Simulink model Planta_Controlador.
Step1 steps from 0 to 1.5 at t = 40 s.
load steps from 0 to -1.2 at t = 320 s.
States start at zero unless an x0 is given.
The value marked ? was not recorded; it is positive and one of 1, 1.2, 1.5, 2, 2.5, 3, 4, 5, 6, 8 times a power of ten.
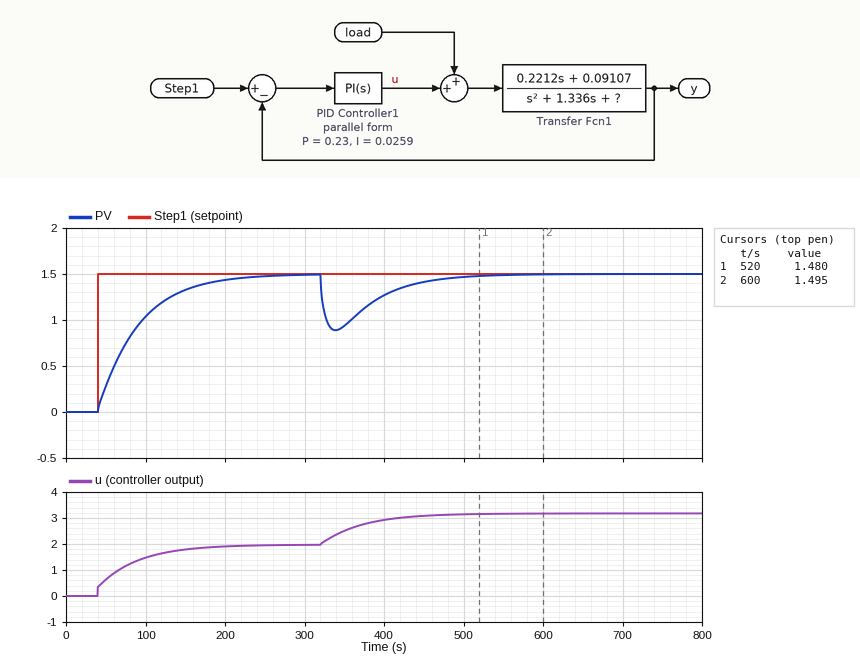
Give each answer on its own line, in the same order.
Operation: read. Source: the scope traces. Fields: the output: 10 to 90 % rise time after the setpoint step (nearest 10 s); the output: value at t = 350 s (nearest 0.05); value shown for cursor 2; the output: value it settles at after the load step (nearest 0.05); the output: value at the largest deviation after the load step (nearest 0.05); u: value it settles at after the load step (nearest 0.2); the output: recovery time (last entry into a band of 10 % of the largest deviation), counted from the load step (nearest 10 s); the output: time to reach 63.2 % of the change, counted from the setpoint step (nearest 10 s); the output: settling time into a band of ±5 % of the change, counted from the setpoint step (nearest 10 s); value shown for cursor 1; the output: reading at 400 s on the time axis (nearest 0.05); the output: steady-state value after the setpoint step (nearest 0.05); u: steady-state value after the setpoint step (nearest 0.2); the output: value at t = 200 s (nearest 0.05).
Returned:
110 s
0.95
1.495
1.50
0.90
3.2
150 s
50 s
150 s
1.480
1.25
1.50
2.0
1.45
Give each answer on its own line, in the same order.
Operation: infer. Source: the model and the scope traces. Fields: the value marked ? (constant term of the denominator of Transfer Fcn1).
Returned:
0.12
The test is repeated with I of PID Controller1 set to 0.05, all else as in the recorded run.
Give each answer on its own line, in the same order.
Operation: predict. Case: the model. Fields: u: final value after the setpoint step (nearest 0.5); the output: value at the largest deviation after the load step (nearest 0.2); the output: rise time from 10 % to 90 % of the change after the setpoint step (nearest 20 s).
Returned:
2.0
1.0
60 s
